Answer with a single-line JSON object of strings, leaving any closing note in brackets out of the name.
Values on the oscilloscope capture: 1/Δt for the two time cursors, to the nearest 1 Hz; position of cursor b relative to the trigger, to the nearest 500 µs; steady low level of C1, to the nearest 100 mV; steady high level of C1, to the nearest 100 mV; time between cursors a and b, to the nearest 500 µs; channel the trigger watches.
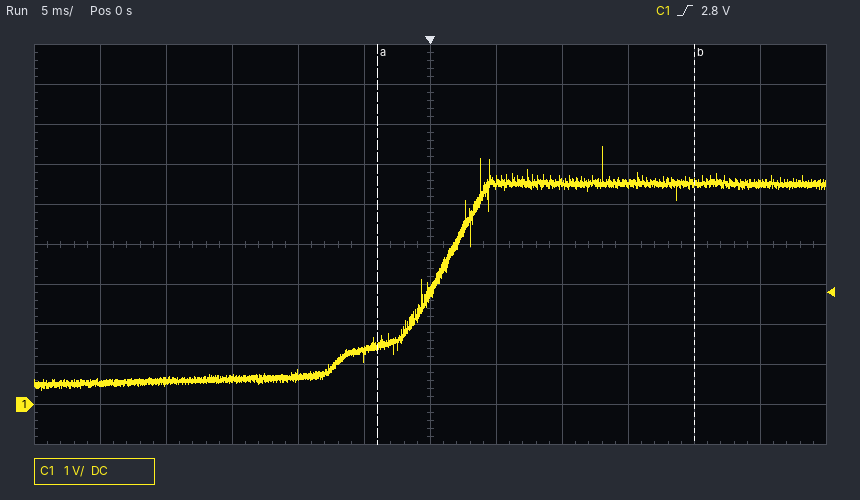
{"1/Δt for the two time cursors, to the nearest 1 Hz": "42 Hz", "position of cursor b relative to the trigger, to the nearest 500 µs": "+20.0 ms", "steady low level of C1, to the nearest 100 mV": "600 mV", "steady high level of C1, to the nearest 100 mV": "5.5 V", "time between cursors a and b, to the nearest 500 µs": "24.0 ms", "channel the trigger watches": "C1"}
